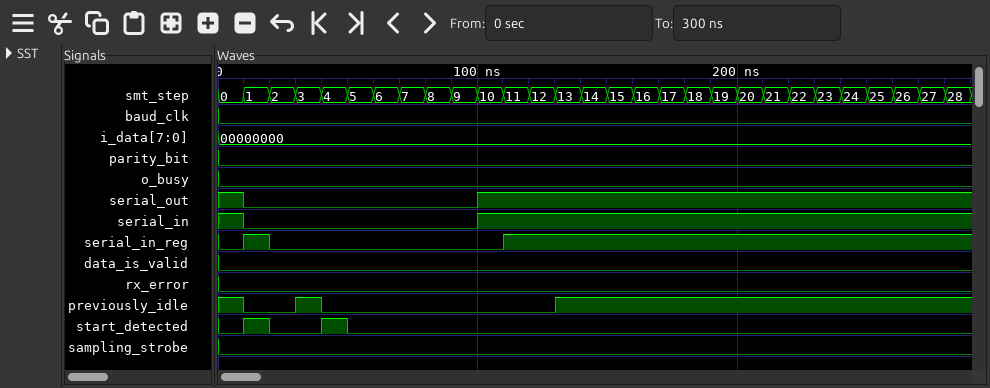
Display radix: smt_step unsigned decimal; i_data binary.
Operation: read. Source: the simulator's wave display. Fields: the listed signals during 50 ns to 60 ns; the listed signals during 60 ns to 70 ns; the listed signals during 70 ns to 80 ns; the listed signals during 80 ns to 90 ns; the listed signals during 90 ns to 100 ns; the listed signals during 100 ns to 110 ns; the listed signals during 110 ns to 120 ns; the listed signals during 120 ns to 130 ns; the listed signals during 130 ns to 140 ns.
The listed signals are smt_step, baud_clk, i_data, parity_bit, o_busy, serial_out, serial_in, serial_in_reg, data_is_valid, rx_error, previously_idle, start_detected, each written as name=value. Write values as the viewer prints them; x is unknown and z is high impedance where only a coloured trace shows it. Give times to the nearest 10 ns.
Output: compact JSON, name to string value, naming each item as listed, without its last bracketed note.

{"the listed signals during 50 ns to 60 ns": "smt_step=5, baud_clk=0, i_data=00000000, parity_bit=0, o_busy=0, serial_out=0, serial_in=0, serial_in_reg=0, data_is_valid=0, rx_error=0, previously_idle=0, start_detected=0", "the listed signals during 60 ns to 70 ns": "smt_step=6, baud_clk=0, i_data=00000000, parity_bit=0, o_busy=0, serial_out=0, serial_in=0, serial_in_reg=0, data_is_valid=0, rx_error=0, previously_idle=0, start_detected=0", "the listed signals during 70 ns to 80 ns": "smt_step=7, baud_clk=0, i_data=00000000, parity_bit=0, o_busy=0, serial_out=0, serial_in=0, serial_in_reg=0, data_is_valid=0, rx_error=0, previously_idle=0, start_detected=0", "the listed signals during 80 ns to 90 ns": "smt_step=8, baud_clk=0, i_data=00000000, parity_bit=0, o_busy=0, serial_out=0, serial_in=0, serial_in_reg=0, data_is_valid=0, rx_error=0, previously_idle=0, start_detected=0", "the listed signals during 90 ns to 100 ns": "smt_step=9, baud_clk=0, i_data=00000000, parity_bit=0, o_busy=0, serial_out=0, serial_in=0, serial_in_reg=0, data_is_valid=0, rx_error=0, previously_idle=0, start_detected=0", "the listed signals during 100 ns to 110 ns": "smt_step=10, baud_clk=0, i_data=00000000, parity_bit=0, o_busy=0, serial_out=1, serial_in=1, serial_in_reg=0, data_is_valid=0, rx_error=0, previously_idle=0, start_detected=0", "the listed signals during 110 ns to 120 ns": "smt_step=11, baud_clk=0, i_data=00000000, parity_bit=0, o_busy=0, serial_out=1, serial_in=1, serial_in_reg=1, data_is_valid=0, rx_error=0, previously_idle=0, start_detected=0", "the listed signals during 120 ns to 130 ns": "smt_step=12, baud_clk=0, i_data=00000000, parity_bit=0, o_busy=0, serial_out=1, serial_in=1, serial_in_reg=1, data_is_valid=0, rx_error=0, previously_idle=0, start_detected=0", "the listed signals during 130 ns to 140 ns": "smt_step=13, baud_clk=0, i_data=00000000, parity_bit=0, o_busy=0, serial_out=1, serial_in=1, serial_in_reg=1, data_is_valid=0, rx_error=0, previously_idle=1, start_detected=0"}
